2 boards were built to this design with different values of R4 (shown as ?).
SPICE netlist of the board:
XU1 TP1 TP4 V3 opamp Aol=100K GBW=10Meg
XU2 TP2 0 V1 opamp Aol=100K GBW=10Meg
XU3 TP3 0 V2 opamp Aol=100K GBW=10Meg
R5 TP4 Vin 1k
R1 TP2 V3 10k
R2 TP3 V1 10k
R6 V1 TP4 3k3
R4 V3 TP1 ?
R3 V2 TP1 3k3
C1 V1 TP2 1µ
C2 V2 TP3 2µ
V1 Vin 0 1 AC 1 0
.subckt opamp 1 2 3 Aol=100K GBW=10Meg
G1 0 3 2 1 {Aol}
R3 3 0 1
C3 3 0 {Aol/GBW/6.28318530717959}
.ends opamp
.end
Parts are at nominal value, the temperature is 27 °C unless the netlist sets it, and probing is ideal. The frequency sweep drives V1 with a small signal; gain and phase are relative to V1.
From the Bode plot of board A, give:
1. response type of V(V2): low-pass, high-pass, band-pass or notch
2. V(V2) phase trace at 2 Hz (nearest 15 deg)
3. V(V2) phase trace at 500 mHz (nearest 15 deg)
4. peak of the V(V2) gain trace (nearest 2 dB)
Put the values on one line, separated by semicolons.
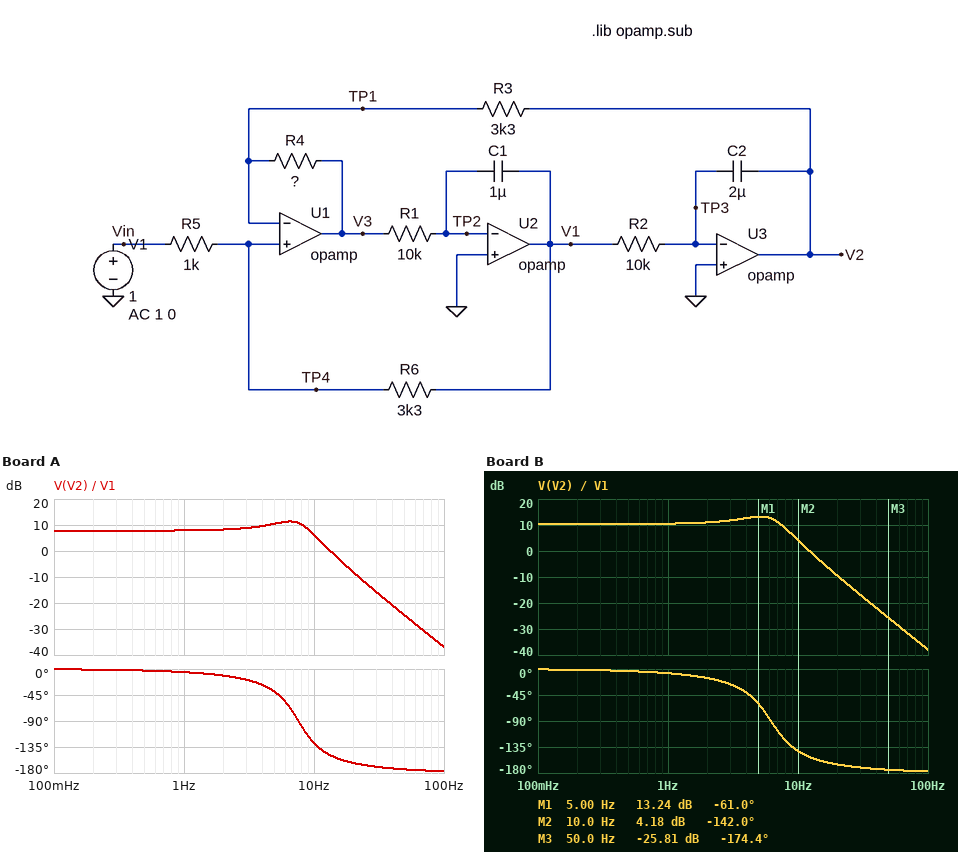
low-pass; -15 deg; 0 deg; 12 dB
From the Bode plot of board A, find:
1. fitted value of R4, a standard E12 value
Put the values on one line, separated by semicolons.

1.5 kΩ
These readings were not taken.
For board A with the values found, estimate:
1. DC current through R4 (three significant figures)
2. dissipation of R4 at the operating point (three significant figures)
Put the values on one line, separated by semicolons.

512 µA; 393 µW
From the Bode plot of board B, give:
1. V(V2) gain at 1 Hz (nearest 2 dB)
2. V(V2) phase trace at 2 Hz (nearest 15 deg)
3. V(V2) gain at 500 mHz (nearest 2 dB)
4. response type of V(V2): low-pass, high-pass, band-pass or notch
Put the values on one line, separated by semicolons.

10 dB; -15 deg; 10 dB; low-pass
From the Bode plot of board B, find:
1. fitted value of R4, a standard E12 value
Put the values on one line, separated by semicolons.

1 kΩ
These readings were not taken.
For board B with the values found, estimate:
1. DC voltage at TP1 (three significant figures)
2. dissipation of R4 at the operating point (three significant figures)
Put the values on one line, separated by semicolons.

767 mV; 589 µW
